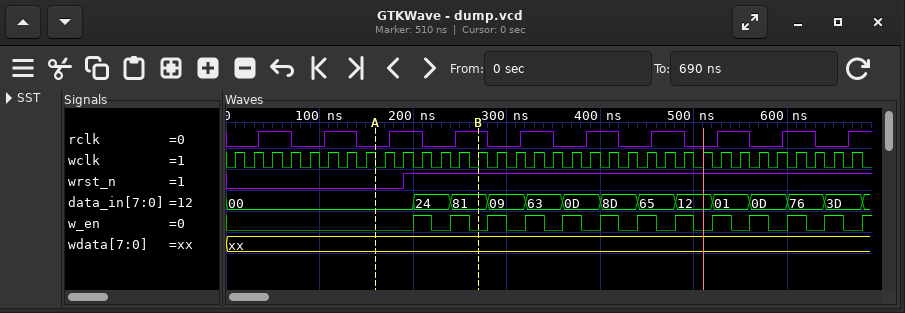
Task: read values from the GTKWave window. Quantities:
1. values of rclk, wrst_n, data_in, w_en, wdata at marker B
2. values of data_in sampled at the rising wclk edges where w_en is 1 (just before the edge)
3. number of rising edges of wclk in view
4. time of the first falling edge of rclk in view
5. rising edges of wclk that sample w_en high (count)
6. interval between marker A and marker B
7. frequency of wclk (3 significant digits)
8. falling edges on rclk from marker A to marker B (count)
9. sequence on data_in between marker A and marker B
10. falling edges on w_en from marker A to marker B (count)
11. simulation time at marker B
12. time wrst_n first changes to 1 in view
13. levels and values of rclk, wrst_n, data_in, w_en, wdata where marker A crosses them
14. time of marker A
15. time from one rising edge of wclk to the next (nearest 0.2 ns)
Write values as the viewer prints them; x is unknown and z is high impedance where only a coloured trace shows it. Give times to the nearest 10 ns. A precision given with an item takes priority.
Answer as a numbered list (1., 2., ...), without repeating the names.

1. rclk=1, wrst_n=1, data_in=81, w_en=0, wdata=xx
2. 24, 81, 09, 63, 0D, 8D, 65, 12, 01, 0D, 76, 3D
3. 34
4. 70 ns
5. 12
6. 110 ns
7. 50.0 MHz
8. 1
9. 00, 24, 81
10. 2
11. 270 ns
12. 190 ns
13. rclk=0, wrst_n=0, data_in=00, w_en=0, wdata=xx
14. 160 ns
15. 20 ns
